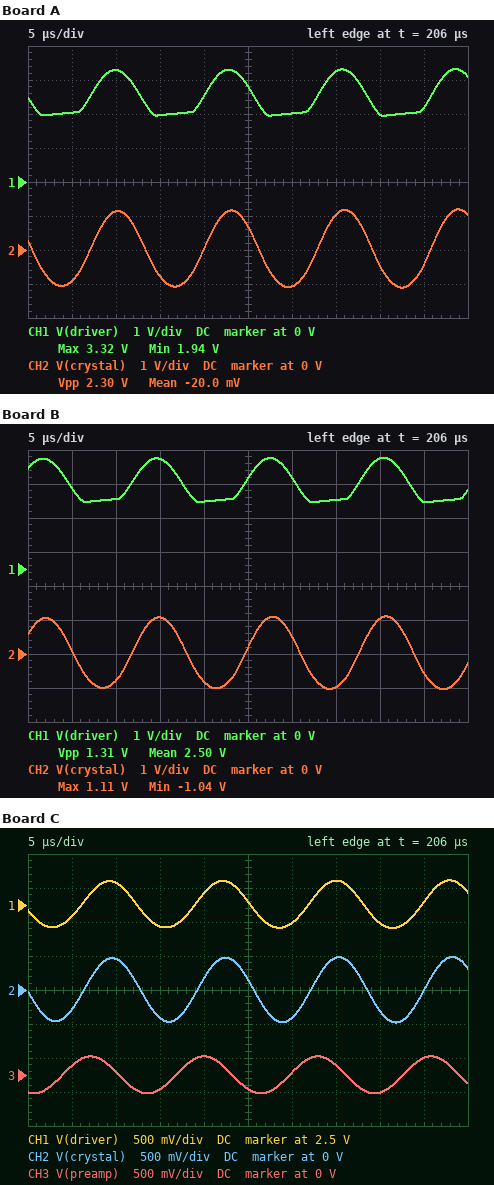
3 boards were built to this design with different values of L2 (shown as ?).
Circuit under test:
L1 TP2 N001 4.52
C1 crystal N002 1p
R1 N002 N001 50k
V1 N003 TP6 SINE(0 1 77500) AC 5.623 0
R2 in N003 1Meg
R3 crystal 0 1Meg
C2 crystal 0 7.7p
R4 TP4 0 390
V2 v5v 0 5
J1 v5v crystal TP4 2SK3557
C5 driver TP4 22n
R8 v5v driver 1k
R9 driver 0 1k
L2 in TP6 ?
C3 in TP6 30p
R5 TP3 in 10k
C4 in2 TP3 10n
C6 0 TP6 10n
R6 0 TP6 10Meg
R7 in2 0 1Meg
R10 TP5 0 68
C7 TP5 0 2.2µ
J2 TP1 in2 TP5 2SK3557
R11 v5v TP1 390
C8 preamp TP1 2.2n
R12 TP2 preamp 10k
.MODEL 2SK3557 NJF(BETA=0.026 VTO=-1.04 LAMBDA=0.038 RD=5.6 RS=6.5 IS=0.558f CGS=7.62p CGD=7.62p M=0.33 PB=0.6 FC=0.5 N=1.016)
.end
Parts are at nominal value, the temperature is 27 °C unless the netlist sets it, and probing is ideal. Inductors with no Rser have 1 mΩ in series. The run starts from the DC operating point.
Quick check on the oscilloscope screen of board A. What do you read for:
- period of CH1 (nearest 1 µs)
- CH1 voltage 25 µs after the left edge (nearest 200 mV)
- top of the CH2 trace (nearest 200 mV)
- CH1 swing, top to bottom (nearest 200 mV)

13 µs
2.8 V
1.2 V
1.4 V
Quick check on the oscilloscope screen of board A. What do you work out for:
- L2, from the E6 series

47 mH
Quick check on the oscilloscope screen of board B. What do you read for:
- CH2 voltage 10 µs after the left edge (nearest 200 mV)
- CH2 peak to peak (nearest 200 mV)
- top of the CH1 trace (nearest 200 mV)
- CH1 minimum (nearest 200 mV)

-800 mV
2.2 V
3.2 V
2.0 V
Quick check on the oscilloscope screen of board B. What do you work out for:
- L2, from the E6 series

100 mH
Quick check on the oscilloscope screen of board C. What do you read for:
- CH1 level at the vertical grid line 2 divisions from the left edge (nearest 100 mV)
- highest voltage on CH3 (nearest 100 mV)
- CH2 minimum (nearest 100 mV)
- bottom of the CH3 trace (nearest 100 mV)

2.8 V
300 mV
-500 mV
-300 mV
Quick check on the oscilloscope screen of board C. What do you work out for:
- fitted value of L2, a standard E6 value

33 mH
